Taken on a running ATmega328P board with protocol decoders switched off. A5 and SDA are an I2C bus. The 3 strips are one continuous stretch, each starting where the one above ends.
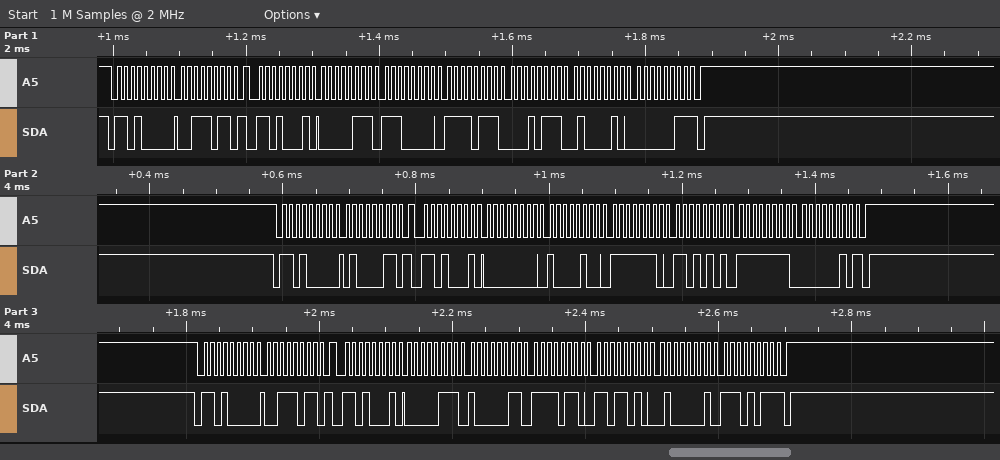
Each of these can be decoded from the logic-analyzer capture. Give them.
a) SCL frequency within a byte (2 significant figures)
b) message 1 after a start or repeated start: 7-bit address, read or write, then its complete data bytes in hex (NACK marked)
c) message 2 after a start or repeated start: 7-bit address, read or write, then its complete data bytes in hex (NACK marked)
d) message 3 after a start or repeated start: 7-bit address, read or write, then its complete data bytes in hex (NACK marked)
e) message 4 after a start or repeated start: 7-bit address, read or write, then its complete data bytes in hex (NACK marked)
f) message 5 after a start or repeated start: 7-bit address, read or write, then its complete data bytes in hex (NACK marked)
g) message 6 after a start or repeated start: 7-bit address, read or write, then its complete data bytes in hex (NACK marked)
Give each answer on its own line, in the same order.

100 kHz
0x68 write: 3B
0x68 read: 07 E0 F7 17 42 03 NACK
0x68 write: 43
0x68 read: 00 84 FE D5 FF 02 NACK
0x68 write: 3B
0x68 read: 07 83 F6 DA 41 EB NACK
